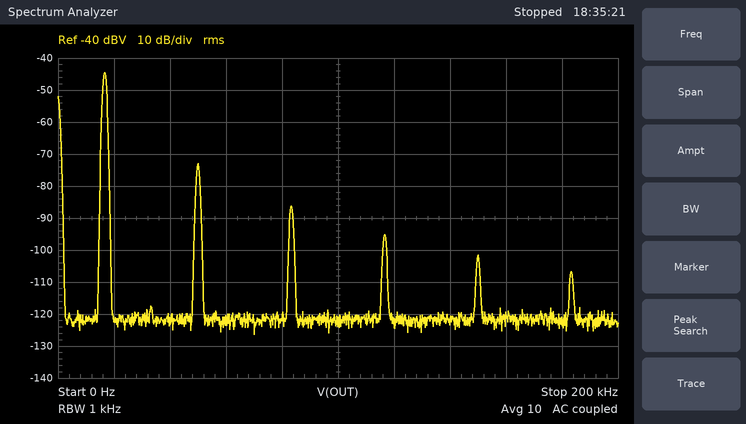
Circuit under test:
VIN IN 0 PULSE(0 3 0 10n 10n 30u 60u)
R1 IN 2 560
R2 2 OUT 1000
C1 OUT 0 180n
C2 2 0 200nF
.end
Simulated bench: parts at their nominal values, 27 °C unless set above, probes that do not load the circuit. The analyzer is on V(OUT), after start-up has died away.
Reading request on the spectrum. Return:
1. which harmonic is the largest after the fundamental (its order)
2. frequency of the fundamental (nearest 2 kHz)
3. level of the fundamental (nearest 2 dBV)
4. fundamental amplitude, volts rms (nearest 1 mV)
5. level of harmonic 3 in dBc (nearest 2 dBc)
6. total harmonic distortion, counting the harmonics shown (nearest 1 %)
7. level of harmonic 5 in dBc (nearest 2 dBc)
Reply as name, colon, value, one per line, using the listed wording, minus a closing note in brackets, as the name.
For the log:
which harmonic is the largest after the fundamental: 3
frequency of the fundamental: 16 kHz
level of the fundamental: -44 dBV
fundamental amplitude, volts rms: 6 mV
level of harmonic 3 in dBc: -28 dBc
total harmonic distortion, counting the harmonics shown: 4 %
level of harmonic 5 in dBc: -42 dBc
